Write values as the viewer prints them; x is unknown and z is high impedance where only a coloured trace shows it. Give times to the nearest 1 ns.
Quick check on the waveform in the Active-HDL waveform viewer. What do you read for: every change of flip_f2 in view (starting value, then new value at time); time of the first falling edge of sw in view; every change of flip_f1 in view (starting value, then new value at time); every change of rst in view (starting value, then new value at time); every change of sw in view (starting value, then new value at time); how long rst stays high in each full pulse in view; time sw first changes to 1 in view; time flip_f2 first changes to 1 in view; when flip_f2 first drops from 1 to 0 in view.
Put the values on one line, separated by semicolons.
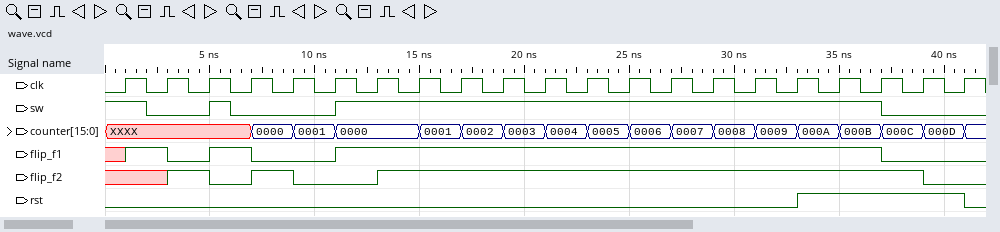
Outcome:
x, 1 at 3 ns, 0 at 5 ns, 1 at 7 ns, 0 at 9 ns, 1 at 13 ns, 0 at 39 ns; 2 ns; x, 1 at 1 ns, 0 at 3 ns, 1 at 5 ns, 0 at 7 ns, 1 at 11 ns, 0 at 37 ns; 0, 1 at 33 ns, 0 at 41 ns; 1, 0 at 2 ns, 1 at 5 ns, 0 at 6 ns, 1 at 11 ns, 0 at 37 ns; 8 ns; 5 ns; 3 ns; 5 ns
